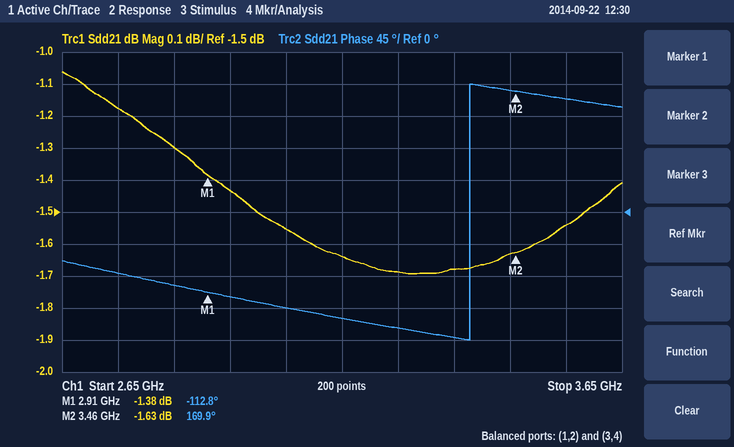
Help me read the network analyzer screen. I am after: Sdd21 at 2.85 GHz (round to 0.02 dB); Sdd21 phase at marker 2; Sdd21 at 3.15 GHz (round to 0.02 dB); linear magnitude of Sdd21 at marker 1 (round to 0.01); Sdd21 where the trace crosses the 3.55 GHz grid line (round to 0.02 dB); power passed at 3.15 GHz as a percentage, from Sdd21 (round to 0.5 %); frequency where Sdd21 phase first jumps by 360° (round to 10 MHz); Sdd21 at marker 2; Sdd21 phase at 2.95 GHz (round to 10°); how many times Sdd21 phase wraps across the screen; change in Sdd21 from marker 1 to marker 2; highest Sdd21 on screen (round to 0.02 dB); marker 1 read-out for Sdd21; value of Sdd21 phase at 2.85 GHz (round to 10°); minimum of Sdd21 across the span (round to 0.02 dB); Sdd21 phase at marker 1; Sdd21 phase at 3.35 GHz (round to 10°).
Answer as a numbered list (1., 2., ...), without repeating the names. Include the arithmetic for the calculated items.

1. -1.30 dB
2. 169.9°
3. -1.64 dB
4. 10^(-1.38/20) ≈ 0.85
5. -1.54 dB
6. 10^(-1.64/10) ≈ 68.5 %
7. 3.38 GHz
8. -1.63 dB
9. -120°
10. 1
11. -1.63 − (-1.38) = -0.25 dB
12. -1.06 dB
13. -1.38 dB
14. -100°
15. -1.70 dB
16. -112.8°
17. -180°
